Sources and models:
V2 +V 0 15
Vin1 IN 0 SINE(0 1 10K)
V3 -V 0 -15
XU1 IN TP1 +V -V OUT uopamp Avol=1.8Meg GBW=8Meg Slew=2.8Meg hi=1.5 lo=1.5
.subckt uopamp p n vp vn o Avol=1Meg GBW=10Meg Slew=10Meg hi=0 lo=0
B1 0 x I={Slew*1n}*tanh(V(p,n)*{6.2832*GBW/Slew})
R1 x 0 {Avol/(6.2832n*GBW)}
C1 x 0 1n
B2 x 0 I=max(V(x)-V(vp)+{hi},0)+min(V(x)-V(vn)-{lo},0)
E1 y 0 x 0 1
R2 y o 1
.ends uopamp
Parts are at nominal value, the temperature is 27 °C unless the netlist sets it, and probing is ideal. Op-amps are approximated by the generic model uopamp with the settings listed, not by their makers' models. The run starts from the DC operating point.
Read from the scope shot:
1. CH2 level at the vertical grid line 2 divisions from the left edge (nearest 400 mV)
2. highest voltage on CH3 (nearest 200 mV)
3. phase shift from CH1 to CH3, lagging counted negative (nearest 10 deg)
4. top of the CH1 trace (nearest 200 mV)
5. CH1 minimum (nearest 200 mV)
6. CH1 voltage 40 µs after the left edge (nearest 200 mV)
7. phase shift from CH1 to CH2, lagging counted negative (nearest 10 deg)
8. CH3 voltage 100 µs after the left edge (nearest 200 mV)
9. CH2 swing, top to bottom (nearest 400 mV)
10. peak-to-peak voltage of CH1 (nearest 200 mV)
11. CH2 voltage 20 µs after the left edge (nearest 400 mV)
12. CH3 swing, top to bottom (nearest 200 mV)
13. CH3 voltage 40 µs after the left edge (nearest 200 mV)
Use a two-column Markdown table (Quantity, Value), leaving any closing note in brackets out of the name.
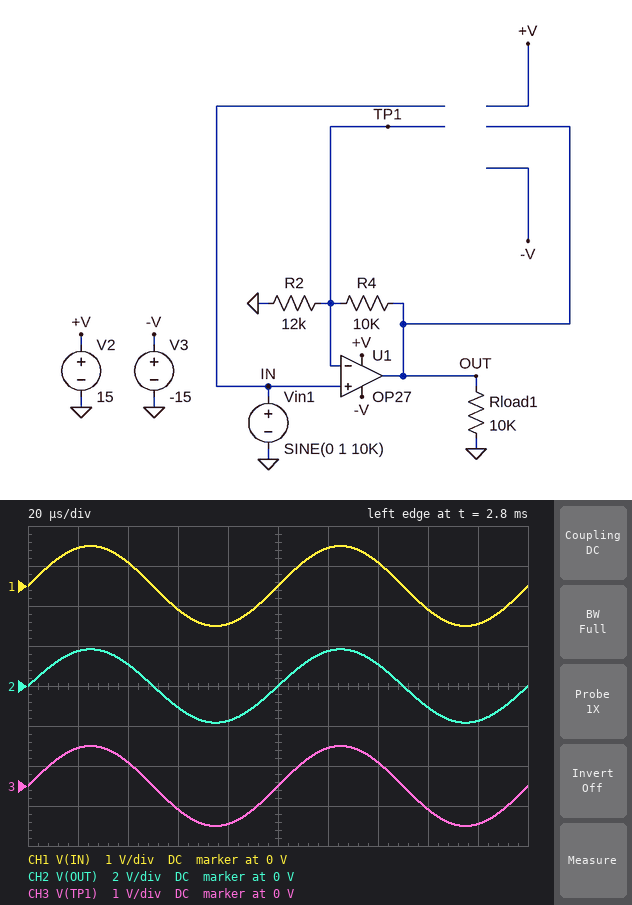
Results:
| Quantity | Value |
|---|---|
| CH2 level at the vertical grid line 2 divisions from the left edge | 1.2 V |
| highest voltage on CH3 | 1.0 V |
| phase shift from CH1 to CH3, lagging counted negative | 0 deg |
| top of the CH1 trace | 1.0 V |
| CH1 minimum | -1.0 V |
| CH1 voltage 40 µs after the left edge | 600 mV |
| phase shift from CH1 to CH2, lagging counted negative | 0 deg |
| CH3 voltage 100 µs after the left edge | 0 V |
| CH2 swing, top to bottom | 3.6 V |
| peak-to-peak voltage of CH1 | 2.0 V |
| CH2 voltage 20 µs after the left edge | 1.6 V |
| CH3 swing, top to bottom | 2.0 V |
| CH3 voltage 40 µs after the left edge | 600 mV |
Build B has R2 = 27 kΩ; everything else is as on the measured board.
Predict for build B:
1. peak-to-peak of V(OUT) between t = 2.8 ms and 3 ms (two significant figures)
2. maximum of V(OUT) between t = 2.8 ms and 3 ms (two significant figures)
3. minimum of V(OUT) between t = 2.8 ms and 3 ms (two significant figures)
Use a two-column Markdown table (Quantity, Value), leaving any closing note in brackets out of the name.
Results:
| Quantity | Value |
|---|---|
| peak-to-peak of V(OUT) between t = 2.8 ms and 3 ms | 2.7 V |
| maximum of V(OUT) between t = 2.8 ms and 3 ms | 1.4 V |
| minimum of V(OUT) between t = 2.8 ms and 3 ms | -1.4 V |
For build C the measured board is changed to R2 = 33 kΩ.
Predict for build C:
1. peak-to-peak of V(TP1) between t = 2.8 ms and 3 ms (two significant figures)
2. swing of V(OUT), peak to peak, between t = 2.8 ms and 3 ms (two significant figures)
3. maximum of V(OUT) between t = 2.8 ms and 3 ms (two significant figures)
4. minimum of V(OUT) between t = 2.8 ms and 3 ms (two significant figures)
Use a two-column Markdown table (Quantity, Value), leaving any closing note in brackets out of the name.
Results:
| Quantity | Value |
|---|---|
| peak-to-peak of V(TP1) between t = 2.8 ms and 3 ms | 2.0 V |
| swing of V(OUT), peak to peak, between t = 2.8 ms and 3 ms | 2.6 V |
| maximum of V(OUT) between t = 2.8 ms and 3 ms | 1.3 V |
| minimum of V(OUT) between t = 2.8 ms and 3 ms | -1.3 V |
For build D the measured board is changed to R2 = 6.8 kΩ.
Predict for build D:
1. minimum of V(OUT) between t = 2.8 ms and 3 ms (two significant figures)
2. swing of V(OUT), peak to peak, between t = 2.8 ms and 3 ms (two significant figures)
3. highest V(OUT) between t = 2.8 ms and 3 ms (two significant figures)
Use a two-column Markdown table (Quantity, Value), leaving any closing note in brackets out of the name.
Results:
| Quantity | Value |
|---|---|
| minimum of V(OUT) between t = 2.8 ms and 3 ms | -2.5 V |
| swing of V(OUT), peak to peak, between t = 2.8 ms and 3 ms | 4.9 V |
| highest V(OUT) between t = 2.8 ms and 3 ms | 2.5 V |
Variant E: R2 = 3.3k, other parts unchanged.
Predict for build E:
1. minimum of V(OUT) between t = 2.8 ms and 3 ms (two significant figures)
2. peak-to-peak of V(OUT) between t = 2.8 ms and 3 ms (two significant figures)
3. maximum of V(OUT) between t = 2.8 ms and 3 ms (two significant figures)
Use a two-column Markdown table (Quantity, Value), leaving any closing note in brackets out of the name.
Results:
| Quantity | Value |
|---|---|
| minimum of V(OUT) between t = 2.8 ms and 3 ms | -4.0 V |
| peak-to-peak of V(OUT) between t = 2.8 ms and 3 ms | 8.1 V |
| maximum of V(OUT) between t = 2.8 ms and 3 ms | 4.0 V |
